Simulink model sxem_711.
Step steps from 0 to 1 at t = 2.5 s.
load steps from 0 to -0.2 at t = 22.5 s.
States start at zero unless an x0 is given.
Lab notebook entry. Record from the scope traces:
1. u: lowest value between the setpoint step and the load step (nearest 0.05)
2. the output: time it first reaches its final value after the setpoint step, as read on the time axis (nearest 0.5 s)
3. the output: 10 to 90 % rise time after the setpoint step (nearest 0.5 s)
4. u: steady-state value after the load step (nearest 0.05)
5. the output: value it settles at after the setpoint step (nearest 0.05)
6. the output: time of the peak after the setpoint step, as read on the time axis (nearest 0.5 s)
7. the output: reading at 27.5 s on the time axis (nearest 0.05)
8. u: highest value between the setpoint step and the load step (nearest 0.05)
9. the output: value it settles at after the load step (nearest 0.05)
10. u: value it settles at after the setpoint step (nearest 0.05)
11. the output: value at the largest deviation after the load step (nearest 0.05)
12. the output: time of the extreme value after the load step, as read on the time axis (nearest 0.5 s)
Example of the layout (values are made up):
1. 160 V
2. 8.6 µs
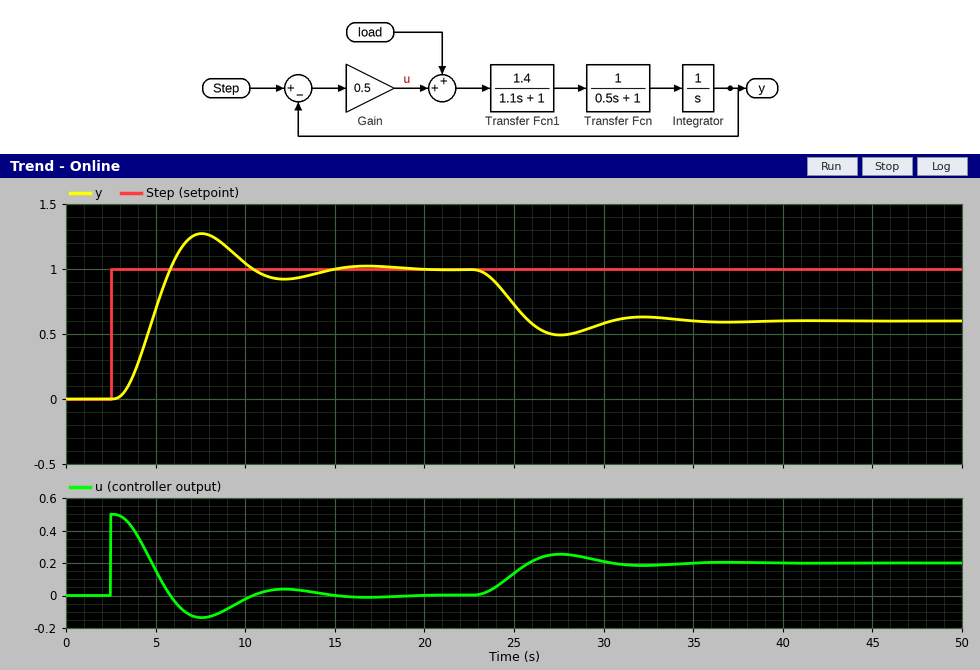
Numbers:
1. -0.15
2. 6.0 s
3. 2.0 s
4. 0.20
5. 1.00
6. 7.5 s
7. 0.50
8. 0.50
9. 0.60
10. 0.00
11. 0.50
12. 27.5 s
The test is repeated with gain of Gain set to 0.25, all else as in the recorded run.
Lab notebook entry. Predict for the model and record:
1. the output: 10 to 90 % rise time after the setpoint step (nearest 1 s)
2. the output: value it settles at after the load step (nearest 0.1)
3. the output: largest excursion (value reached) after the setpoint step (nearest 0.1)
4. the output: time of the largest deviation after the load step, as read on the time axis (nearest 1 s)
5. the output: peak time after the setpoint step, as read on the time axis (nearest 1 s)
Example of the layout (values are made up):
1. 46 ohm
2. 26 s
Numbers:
1. 4 s
2. 0.2
3. 1.1
4. 31 s
5. 11 s
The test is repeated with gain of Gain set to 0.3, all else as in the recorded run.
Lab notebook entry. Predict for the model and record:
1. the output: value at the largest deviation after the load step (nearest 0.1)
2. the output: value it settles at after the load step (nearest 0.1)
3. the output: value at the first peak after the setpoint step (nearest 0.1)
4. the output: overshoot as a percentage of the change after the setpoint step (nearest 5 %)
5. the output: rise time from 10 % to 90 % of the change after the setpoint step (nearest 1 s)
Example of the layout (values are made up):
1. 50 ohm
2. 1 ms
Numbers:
1. 0.3
2. 0.3
3. 1.1
4. 10 %
5. 3 s
